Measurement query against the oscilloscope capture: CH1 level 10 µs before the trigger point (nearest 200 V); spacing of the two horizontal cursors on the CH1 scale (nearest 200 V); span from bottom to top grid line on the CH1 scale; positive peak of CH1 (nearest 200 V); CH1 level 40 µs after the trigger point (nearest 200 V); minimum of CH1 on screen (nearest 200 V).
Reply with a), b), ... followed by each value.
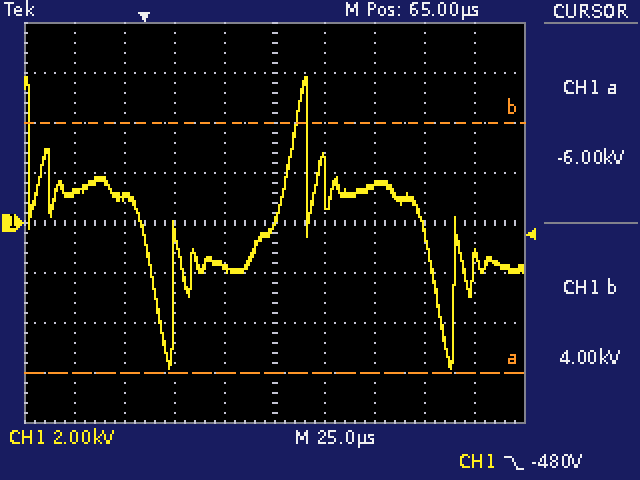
a) 1.0 kV
b) 10.0 kV
c) 16 kV
d) 5.8 kV
e) -1.8 kV
f) -5.8 kV
